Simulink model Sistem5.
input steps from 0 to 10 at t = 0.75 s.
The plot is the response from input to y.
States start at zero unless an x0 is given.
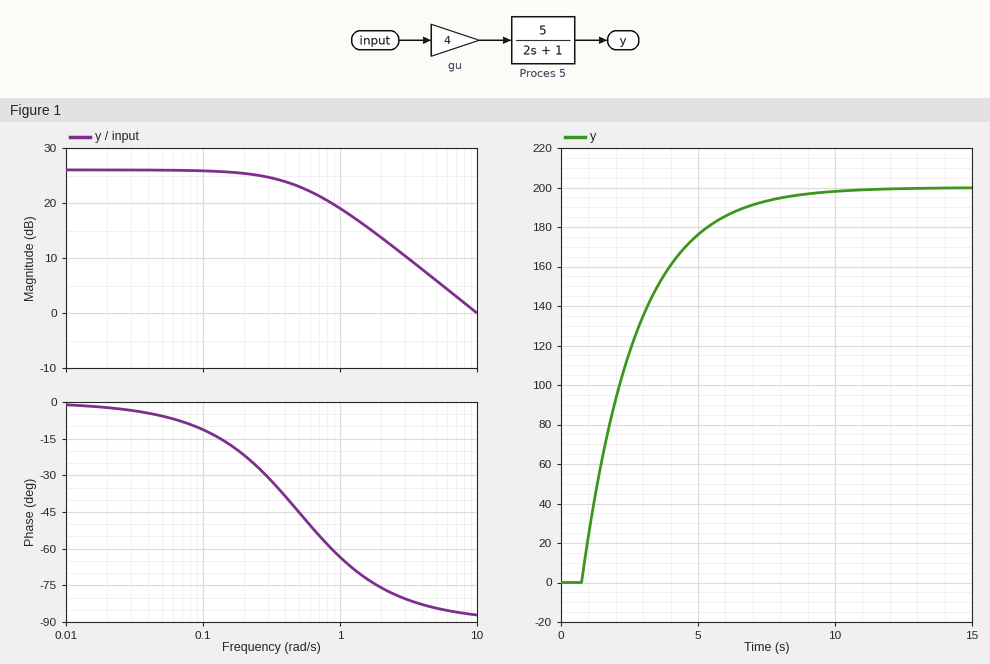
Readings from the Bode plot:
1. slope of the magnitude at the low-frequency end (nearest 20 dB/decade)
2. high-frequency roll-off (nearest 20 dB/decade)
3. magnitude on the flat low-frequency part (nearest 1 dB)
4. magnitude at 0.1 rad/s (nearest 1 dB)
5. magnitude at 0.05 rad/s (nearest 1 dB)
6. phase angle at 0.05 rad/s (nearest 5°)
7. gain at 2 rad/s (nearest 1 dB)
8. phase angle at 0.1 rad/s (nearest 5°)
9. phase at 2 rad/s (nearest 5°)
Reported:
0 dB/decade
-20 dB/decade
26 dB
26 dB
26 dB
-5°
14 dB
-10°
-75°
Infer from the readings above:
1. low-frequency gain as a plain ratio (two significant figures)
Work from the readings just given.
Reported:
20
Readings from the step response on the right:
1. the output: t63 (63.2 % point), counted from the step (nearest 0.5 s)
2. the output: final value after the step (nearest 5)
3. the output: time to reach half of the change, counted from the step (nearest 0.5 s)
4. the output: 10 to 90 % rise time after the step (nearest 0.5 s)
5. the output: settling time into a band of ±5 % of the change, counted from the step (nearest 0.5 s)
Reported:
2.0 s
200
1.5 s
4.5 s
6.0 s
